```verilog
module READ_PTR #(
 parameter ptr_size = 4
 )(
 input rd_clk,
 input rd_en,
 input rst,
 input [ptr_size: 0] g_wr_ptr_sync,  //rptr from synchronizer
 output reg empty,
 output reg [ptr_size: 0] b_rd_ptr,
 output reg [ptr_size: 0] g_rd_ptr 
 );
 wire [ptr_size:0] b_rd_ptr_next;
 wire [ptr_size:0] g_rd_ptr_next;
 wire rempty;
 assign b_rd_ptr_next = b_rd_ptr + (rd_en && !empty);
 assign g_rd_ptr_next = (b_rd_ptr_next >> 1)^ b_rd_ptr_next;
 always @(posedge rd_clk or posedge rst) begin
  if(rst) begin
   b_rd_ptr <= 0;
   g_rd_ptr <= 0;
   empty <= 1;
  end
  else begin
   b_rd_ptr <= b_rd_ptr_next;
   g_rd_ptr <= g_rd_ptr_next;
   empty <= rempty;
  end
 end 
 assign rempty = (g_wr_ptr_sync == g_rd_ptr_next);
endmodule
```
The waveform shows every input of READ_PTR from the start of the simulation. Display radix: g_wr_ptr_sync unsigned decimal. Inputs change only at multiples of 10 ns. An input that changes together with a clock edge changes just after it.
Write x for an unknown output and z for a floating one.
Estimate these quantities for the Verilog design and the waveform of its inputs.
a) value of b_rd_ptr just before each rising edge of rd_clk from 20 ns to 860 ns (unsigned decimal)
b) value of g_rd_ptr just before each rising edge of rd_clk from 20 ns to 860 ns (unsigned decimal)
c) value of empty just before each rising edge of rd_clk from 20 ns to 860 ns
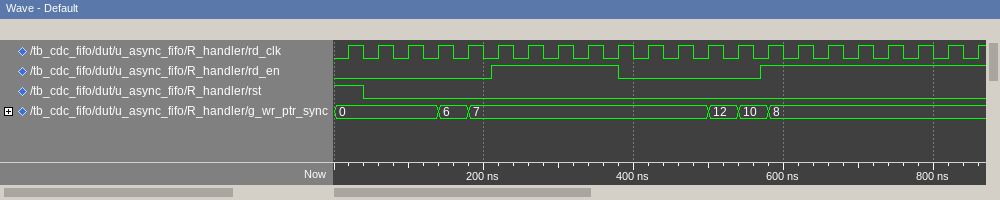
0, 0, 0, 0, 0, 0, 1, 2, 3, 4, 5, 5, 5, 5, 5, 6, 7, 8, 9, 10, 11, 12
0, 0, 0, 0, 0, 0, 1, 3, 2, 6, 7, 7, 7, 7, 7, 5, 4, 12, 13, 15, 14, 10
1 1 1 1 1 0 0 0 0 0 1 1 1 1 0 0 0 0 0 0 0 0
